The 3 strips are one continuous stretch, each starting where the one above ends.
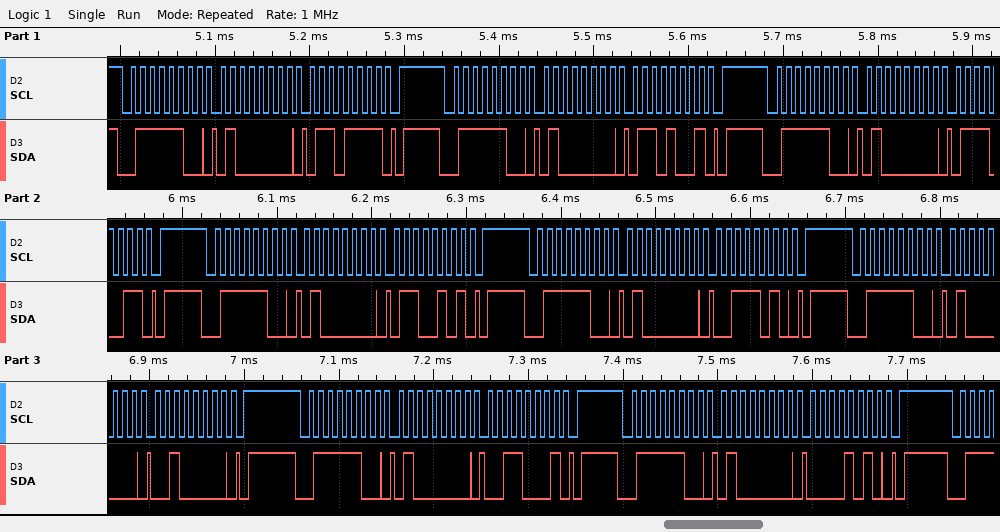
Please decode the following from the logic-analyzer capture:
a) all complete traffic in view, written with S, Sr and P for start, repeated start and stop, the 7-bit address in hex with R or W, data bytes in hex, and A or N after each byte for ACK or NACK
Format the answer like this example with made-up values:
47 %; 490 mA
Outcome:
S 3EW A 40 A 6F A P S 3EW A 40 A 69 A P S 3EW A 40 A 73 A P S 3EW A 40 A 65 A P S 3EW A 40 A 3A A P S 3EW A 40 A 20 A P S 3EW A 40 A 31 A P S 3EW A 40 A 0A A P
